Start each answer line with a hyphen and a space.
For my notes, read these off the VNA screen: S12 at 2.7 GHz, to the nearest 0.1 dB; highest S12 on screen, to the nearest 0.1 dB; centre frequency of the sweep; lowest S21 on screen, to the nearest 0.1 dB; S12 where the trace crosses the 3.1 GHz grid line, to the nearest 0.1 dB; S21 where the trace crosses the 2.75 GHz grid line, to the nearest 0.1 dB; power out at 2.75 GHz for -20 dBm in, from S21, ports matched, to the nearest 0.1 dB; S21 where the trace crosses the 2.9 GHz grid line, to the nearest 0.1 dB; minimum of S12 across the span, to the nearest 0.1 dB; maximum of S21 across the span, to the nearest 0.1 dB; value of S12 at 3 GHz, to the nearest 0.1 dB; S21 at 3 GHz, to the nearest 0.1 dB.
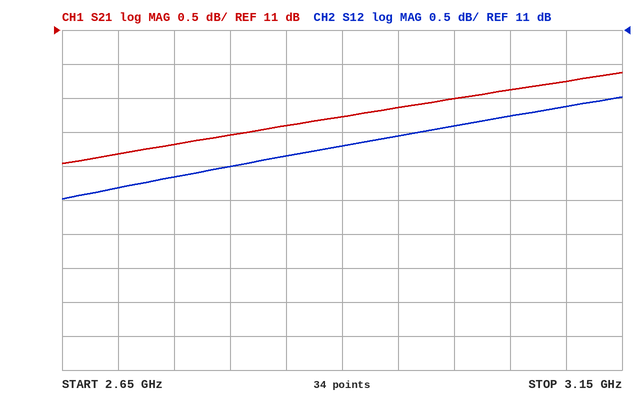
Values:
- 8.7 dB
- 10.0 dB
- 2.9 GHz
- 9.0 dB
- 9.9 dB
- 9.3 dB
- -10.7 dBm
- 9.7 dB
- 8.5 dB
- 10.4 dB
- 9.6 dB
- 10.0 dB
